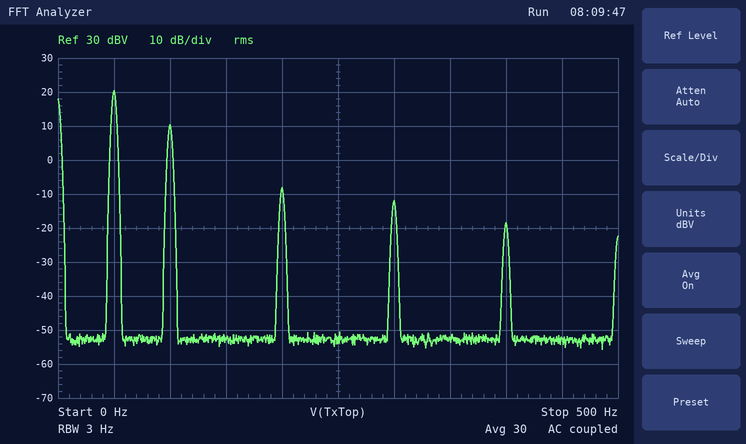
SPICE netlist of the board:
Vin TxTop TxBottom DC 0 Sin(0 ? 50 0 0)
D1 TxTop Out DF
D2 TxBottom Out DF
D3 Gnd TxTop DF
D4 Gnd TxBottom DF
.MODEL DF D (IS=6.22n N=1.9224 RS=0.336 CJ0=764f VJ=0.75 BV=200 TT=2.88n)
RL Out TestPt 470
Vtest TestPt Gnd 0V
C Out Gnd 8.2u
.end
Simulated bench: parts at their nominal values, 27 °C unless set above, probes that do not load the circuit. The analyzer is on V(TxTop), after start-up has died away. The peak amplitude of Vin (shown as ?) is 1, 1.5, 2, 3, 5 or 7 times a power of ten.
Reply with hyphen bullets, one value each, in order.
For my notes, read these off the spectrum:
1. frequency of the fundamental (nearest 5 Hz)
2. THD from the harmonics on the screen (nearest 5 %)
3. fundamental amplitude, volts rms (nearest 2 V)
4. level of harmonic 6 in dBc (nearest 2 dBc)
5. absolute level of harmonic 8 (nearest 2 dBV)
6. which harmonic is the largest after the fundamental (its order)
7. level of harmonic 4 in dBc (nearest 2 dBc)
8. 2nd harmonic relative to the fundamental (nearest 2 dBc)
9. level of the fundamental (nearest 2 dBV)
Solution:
- 50 Hz
- 30 %
- 10 V
- -32 dBc
- -18 dBV
- 2
- -28 dBc
- -10 dBc
- 20 dBV
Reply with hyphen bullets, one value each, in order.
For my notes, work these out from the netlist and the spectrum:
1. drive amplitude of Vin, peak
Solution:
- 30 V
